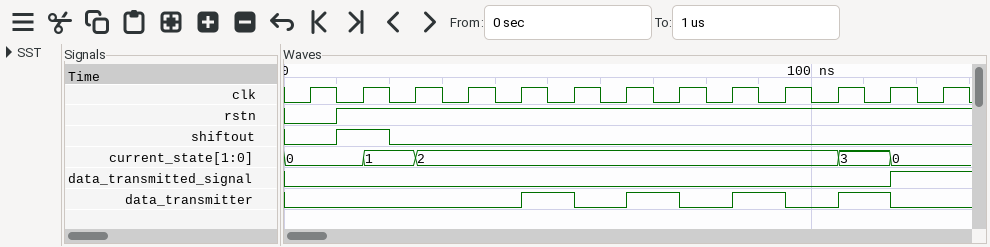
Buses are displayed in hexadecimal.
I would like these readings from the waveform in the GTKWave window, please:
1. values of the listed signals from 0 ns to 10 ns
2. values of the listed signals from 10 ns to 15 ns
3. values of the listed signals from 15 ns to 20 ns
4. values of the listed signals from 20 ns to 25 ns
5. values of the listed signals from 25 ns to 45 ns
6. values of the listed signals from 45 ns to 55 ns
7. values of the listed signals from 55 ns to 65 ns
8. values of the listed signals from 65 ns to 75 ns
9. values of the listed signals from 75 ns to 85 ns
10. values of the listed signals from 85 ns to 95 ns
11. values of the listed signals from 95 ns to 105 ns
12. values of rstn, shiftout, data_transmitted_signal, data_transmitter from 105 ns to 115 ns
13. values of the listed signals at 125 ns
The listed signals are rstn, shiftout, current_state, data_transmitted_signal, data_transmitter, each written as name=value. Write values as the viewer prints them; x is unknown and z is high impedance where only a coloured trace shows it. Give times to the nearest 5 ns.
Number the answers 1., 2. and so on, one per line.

1. rstn=0, shiftout=0, current_state=0, data_transmitted_signal=0, data_transmitter=0
2. rstn=1, shiftout=1, current_state=0, data_transmitted_signal=0, data_transmitter=0
3. rstn=1, shiftout=1, current_state=1, data_transmitted_signal=0, data_transmitter=0
4. rstn=1, shiftout=0, current_state=1, data_transmitted_signal=0, data_transmitter=0
5. rstn=1, shiftout=0, current_state=2, data_transmitted_signal=0, data_transmitter=0
6. rstn=1, shiftout=0, current_state=2, data_transmitted_signal=0, data_transmitter=1
7. rstn=1, shiftout=0, current_state=2, data_transmitted_signal=0, data_transmitter=0
8. rstn=1, shiftout=0, current_state=2, data_transmitted_signal=0, data_transmitter=1
9. rstn=1, shiftout=0, current_state=2, data_transmitted_signal=0, data_transmitter=0
10. rstn=1, shiftout=0, current_state=2, data_transmitted_signal=0, data_transmitter=1
11. rstn=1, shiftout=0, current_state=2, data_transmitted_signal=0, data_transmitter=0
12. rstn=1, shiftout=0, data_transmitted_signal=0, data_transmitter=1
13. rstn=1, shiftout=0, current_state=0, data_transmitted_signal=1, data_transmitter=0
